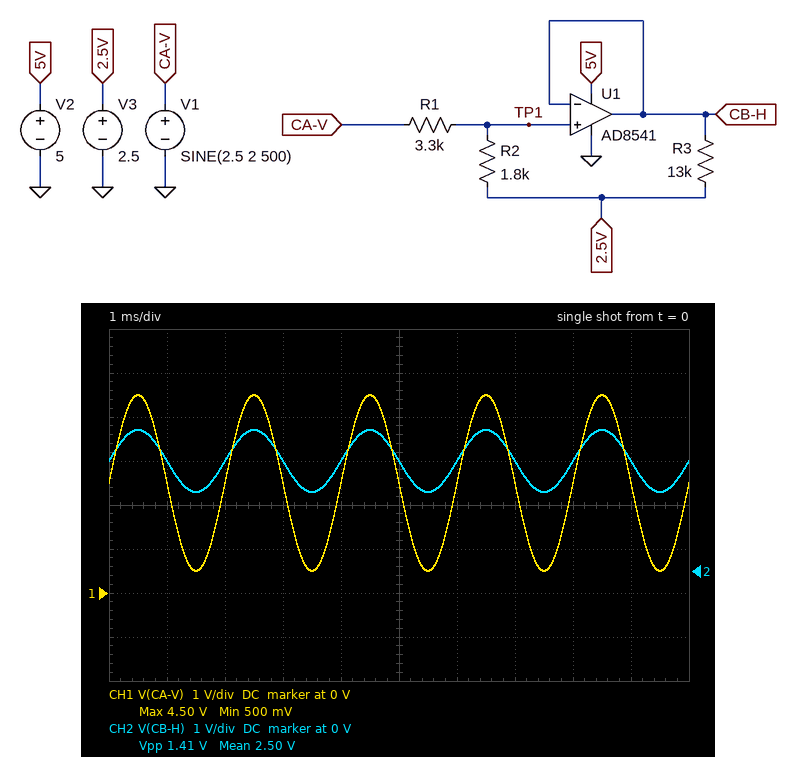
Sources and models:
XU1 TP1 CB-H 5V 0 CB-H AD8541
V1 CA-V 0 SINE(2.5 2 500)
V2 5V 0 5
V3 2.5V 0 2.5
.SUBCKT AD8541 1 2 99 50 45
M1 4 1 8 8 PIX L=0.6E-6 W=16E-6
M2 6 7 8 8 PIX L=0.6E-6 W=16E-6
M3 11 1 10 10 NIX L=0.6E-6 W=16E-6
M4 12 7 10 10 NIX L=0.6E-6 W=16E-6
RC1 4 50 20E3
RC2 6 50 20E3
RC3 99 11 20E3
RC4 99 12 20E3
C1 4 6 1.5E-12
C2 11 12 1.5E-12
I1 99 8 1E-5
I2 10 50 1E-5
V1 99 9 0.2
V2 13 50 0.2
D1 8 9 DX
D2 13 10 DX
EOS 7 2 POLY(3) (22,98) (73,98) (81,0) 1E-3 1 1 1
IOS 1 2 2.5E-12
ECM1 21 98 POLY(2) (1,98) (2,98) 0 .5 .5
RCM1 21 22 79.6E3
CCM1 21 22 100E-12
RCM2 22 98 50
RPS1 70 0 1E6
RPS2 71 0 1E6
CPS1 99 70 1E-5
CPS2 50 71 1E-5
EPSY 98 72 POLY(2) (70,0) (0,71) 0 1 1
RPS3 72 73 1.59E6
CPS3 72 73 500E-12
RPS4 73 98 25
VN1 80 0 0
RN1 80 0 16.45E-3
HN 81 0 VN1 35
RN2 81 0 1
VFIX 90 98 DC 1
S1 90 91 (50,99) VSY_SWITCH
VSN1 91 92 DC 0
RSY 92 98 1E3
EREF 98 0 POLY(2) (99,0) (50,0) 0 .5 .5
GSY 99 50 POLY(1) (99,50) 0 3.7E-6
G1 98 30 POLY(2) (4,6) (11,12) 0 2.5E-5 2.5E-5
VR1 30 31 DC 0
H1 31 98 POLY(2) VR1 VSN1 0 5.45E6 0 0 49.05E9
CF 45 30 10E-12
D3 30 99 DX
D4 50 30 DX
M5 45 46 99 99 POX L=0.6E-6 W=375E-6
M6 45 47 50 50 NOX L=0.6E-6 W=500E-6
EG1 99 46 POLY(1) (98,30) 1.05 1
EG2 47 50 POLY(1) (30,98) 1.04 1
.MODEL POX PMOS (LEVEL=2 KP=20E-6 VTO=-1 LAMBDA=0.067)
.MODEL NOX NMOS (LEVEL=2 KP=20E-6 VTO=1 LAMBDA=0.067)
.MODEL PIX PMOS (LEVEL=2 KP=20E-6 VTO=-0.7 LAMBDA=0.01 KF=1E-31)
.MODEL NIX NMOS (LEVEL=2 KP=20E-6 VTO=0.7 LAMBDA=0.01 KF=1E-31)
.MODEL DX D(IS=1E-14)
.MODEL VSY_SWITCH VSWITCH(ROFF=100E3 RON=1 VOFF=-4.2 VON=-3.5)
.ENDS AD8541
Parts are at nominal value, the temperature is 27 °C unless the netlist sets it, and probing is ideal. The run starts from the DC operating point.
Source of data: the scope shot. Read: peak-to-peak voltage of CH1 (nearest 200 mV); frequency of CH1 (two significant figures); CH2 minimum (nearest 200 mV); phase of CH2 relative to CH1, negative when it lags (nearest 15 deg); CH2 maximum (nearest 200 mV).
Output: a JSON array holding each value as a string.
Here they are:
["4.0 V", "500 Hz", "1.8 V", "0 deg", "3.2 V"]
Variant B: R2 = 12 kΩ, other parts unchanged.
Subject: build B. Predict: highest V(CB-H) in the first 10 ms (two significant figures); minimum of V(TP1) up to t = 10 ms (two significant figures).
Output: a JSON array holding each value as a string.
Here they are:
["4.1 V", "930 mV"]
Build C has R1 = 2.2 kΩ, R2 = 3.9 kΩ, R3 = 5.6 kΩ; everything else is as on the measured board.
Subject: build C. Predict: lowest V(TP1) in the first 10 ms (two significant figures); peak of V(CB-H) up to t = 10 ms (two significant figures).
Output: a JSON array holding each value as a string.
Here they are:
["1.2 V", "3.8 V"]
